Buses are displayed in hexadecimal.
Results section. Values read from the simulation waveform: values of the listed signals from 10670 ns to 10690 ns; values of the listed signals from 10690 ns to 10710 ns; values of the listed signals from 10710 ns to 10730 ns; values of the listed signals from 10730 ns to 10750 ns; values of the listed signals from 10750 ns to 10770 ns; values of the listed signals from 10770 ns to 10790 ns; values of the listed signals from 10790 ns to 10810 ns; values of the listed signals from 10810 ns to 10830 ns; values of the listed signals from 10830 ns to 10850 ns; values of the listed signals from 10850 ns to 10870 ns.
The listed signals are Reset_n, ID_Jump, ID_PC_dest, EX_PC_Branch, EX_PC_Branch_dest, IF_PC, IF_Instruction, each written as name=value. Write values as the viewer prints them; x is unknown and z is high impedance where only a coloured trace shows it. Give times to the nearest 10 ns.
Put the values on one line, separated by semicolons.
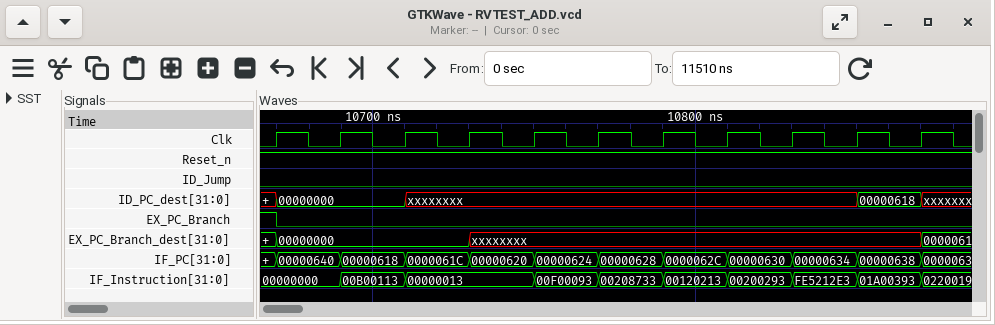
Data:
Reset_n=1, ID_Jump=0, ID_PC_dest=00000000, EX_PC_Branch=0, EX_PC_Branch_dest=00000000, IF_PC=00000640, IF_Instruction=00000000; Reset_n=1, ID_Jump=0, ID_PC_dest=00000000, EX_PC_Branch=0, EX_PC_Branch_dest=00000000, IF_PC=00000618, IF_Instruction=00B00113; Reset_n=1, ID_Jump=0, ID_PC_dest=xxxxxxxx, EX_PC_Branch=0, EX_PC_Branch_dest=00000000, IF_PC=0000061C, IF_Instruction=00000013; Reset_n=1, ID_Jump=0, ID_PC_dest=xxxxxxxx, EX_PC_Branch=0, EX_PC_Branch_dest=xxxxxxxx, IF_PC=00000620, IF_Instruction=00000013; Reset_n=1, ID_Jump=0, ID_PC_dest=xxxxxxxx, EX_PC_Branch=0, EX_PC_Branch_dest=xxxxxxxx, IF_PC=00000624, IF_Instruction=00F00093; Reset_n=1, ID_Jump=0, ID_PC_dest=xxxxxxxx, EX_PC_Branch=0, EX_PC_Branch_dest=xxxxxxxx, IF_PC=00000628, IF_Instruction=00208733; Reset_n=1, ID_Jump=0, ID_PC_dest=xxxxxxxx, EX_PC_Branch=0, EX_PC_Branch_dest=xxxxxxxx, IF_PC=0000062C, IF_Instruction=00120213; Reset_n=1, ID_Jump=0, ID_PC_dest=xxxxxxxx, EX_PC_Branch=0, EX_PC_Branch_dest=xxxxxxxx, IF_PC=00000630, IF_Instruction=00200293; Reset_n=1, ID_Jump=0, ID_PC_dest=xxxxxxxx, EX_PC_Branch=0, EX_PC_Branch_dest=xxxxxxxx, IF_PC=00000634, IF_Instruction=FE5212E3; Reset_n=1, ID_Jump=0, ID_PC_dest=00000618, EX_PC_Branch=0, EX_PC_Branch_dest=xxxxxxxx, IF_PC=00000638, IF_Instruction=01A00393
